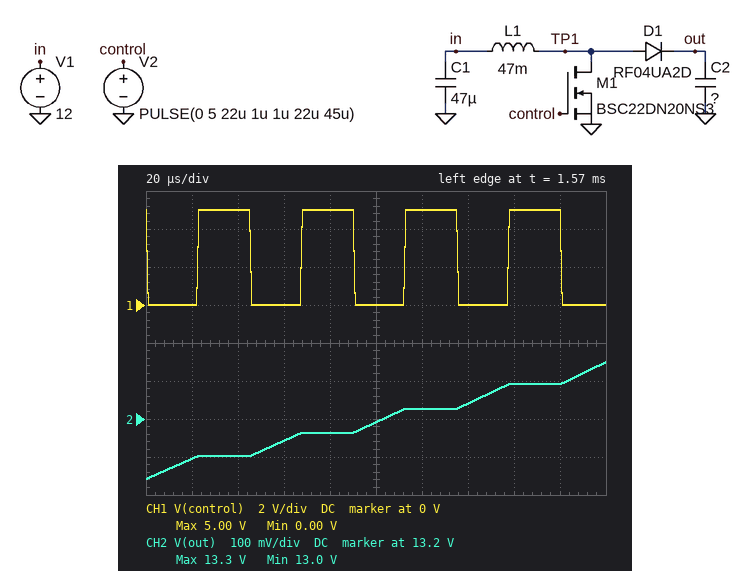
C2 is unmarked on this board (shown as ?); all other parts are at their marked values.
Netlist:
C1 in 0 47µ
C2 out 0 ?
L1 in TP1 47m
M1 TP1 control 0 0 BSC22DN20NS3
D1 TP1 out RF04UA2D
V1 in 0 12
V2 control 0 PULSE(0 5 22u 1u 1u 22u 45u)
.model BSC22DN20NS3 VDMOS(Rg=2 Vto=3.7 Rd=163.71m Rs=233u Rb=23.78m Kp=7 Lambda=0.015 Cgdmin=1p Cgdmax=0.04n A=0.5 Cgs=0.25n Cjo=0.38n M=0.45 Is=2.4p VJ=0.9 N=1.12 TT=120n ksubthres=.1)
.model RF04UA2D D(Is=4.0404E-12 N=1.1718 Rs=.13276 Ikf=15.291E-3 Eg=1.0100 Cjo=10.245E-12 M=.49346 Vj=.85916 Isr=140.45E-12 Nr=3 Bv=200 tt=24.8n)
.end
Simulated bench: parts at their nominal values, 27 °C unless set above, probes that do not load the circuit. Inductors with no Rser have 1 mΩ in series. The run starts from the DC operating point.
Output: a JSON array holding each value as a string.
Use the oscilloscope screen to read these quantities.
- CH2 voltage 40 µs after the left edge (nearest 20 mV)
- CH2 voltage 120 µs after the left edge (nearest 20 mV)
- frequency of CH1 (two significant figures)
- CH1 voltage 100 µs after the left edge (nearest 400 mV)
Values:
["13.10 V", "13.22 V", "22 kHz", "0 V"]
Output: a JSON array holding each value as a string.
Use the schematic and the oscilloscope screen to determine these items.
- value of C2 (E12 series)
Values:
["68 µF"]
